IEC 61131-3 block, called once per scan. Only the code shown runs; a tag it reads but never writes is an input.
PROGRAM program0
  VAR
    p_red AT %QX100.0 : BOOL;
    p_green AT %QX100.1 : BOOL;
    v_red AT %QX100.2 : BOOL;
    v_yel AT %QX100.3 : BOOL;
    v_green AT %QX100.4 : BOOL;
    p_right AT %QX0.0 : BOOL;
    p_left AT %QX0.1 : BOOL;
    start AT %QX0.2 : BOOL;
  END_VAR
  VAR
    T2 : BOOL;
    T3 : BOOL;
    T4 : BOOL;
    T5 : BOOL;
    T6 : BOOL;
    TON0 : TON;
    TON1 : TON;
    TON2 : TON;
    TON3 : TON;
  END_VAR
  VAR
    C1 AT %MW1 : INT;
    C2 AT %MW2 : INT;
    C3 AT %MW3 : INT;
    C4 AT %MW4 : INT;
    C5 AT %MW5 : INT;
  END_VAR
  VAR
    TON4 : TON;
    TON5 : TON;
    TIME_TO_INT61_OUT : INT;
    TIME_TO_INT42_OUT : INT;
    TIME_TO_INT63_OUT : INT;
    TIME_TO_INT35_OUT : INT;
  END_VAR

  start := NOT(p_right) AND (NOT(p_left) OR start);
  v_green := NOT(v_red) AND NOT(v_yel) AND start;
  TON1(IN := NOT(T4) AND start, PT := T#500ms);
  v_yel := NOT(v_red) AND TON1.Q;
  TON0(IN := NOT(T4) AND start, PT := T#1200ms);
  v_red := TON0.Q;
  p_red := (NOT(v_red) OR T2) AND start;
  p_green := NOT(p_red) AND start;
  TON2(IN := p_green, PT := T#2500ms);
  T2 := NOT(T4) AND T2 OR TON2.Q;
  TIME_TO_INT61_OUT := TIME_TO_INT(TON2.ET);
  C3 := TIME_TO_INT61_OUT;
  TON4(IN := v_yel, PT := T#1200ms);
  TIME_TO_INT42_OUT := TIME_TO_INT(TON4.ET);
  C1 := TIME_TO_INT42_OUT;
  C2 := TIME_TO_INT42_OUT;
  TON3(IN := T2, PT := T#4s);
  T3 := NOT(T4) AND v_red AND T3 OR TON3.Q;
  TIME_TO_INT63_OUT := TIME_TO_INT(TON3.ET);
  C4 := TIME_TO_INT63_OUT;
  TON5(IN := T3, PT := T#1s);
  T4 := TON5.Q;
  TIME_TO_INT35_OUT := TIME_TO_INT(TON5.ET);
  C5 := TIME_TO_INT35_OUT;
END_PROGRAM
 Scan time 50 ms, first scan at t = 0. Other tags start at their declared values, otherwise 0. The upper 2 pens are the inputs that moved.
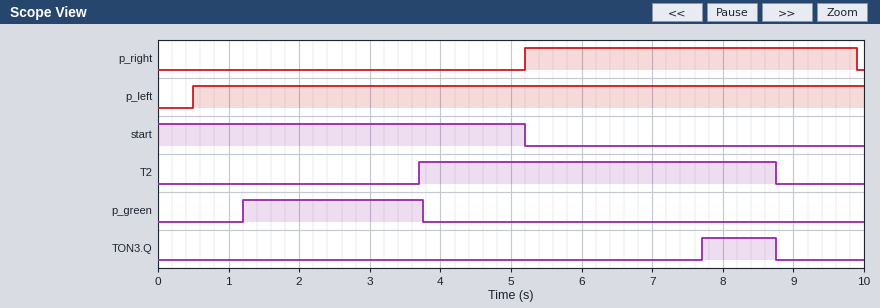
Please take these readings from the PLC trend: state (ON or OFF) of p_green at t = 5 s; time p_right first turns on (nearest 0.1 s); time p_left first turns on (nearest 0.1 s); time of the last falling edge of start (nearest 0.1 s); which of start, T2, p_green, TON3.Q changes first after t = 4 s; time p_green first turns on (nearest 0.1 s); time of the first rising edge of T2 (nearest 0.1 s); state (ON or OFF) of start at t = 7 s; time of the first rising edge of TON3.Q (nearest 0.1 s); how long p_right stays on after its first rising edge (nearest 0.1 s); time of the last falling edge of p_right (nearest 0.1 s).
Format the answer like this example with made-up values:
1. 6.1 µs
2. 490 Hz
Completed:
1. OFF
2. 5.2 s
3. 0.5 s
4. 5.2 s
5. start
6. 1.2 s
7. 3.7 s
8. OFF
9. 7.7 s
10. 4.7 s
11. 9.9 s
